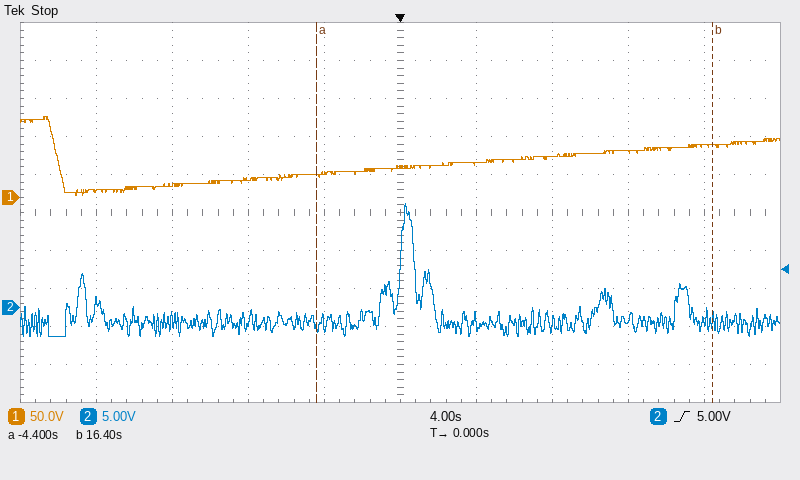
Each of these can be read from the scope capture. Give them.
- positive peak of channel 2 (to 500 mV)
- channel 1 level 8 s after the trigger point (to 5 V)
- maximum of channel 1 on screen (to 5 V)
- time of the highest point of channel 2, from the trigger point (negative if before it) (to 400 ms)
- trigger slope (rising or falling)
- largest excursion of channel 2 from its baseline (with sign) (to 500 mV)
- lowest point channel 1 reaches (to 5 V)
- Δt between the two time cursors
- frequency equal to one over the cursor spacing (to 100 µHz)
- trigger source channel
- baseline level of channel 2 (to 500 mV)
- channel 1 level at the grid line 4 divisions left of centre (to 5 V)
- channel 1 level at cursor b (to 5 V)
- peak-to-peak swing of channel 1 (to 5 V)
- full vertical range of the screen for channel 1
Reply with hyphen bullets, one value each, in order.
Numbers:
- 13.5 V
- 55 V
- 105 V
- +400 ms
- rising
- +15.5 V
- 0 V
- 20.8 s
- 48.1 mHz
- channel 2
- -2.0 V
- 10 V
- 70 V
- 105 V
- 500 V
